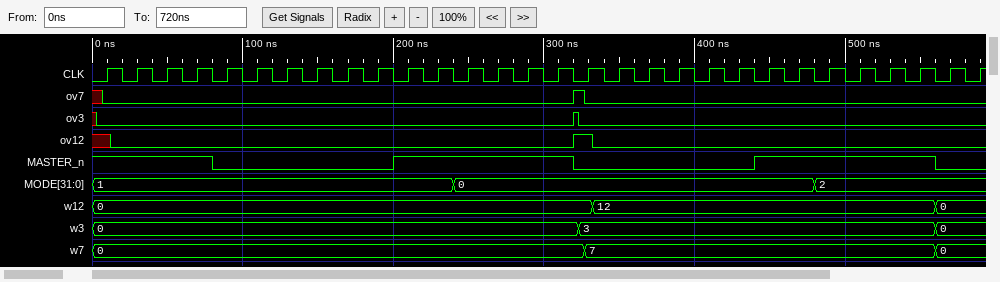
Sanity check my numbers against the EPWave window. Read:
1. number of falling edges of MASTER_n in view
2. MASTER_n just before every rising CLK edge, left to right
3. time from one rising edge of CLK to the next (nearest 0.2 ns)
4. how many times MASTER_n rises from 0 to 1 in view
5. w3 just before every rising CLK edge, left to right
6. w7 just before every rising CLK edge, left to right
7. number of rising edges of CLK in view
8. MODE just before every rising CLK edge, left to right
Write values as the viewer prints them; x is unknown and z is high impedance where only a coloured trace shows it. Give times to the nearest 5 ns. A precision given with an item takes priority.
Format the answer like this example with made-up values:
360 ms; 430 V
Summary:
3; 1 1 1 1 0 0 0 0 0 0 1 1 1 1 1 1 0 0 0 0 0 0 1 1 1 1 1 1 0 0; 20 ns; 2; 0, 0, 0, 0, 0, 0, 0, 0, 0, 0, 0, 0, 0, 0, 0, 0, 3, 3, 3, 3, 3, 3, 3, 3, 3, 3, 3, 3, 0, 0; 0, 0, 0, 0, 0, 0, 0, 0, 0, 0, 0, 0, 0, 0, 0, 0, 7, 7, 7, 7, 7, 7, 7, 7, 7, 7, 7, 7, 0, 0; 30; 1, 1, 1, 1, 1, 1, 1, 1, 1, 1, 1, 1, 0, 0, 0, 0, 0, 0, 0, 0, 0, 0, 0, 0, 2, 2, 2, 2, 2, 2
